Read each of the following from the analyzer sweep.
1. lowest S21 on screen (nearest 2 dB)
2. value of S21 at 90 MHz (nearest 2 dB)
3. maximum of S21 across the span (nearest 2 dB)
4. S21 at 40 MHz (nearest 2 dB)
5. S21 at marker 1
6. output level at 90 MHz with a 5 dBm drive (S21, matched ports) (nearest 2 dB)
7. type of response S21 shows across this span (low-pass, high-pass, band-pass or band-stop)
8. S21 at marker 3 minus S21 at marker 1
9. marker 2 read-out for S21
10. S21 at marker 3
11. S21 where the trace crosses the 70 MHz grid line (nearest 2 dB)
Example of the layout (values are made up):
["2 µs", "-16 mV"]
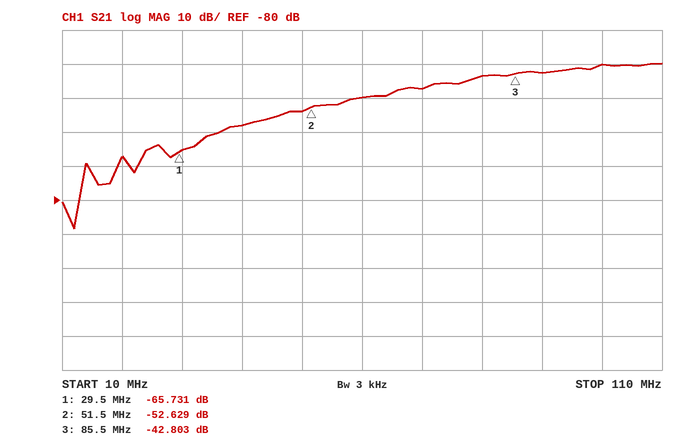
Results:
["-88 dB", "-42 dB", "-40 dB", "-58 dB", "-65.731 dB", "-38 dBm", "high-pass", "22.928 dB", "-52.629 dB", "-42.803 dB", "-48 dB"]
